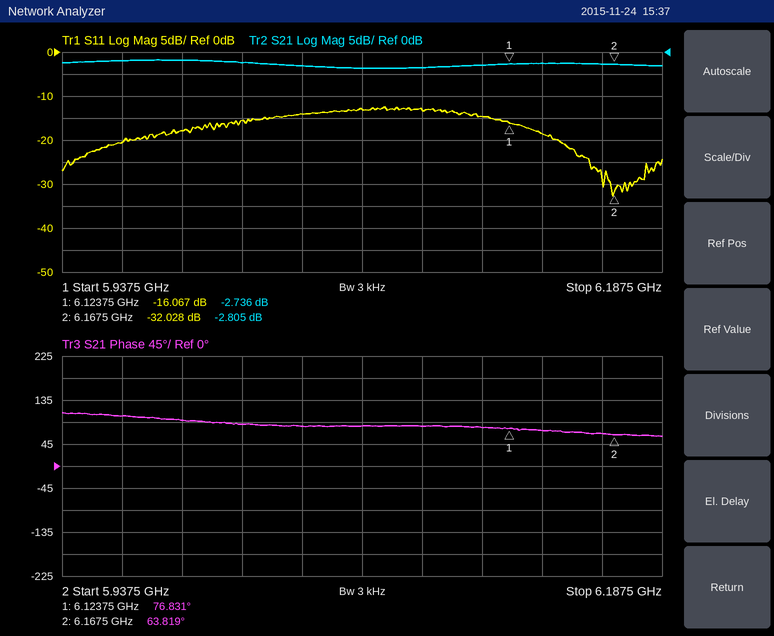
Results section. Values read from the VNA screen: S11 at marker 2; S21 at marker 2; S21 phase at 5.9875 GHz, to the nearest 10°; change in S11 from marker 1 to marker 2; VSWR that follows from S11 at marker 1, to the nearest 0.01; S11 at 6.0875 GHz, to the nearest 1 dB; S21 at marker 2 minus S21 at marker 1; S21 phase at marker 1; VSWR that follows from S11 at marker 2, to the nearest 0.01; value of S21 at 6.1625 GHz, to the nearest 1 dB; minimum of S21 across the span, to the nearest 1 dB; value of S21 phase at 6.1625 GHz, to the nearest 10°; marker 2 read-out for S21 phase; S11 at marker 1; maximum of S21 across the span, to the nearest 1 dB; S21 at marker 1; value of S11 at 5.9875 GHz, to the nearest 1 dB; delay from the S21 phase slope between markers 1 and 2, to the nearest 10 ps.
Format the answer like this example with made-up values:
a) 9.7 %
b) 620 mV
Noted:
a) -32.028 dB
b) -2.805 dB
c) 90°
d) -15.961 dB
e) 1.37
f) -13 dB
g) -0.069 dB
h) 76.831°
i) 1.05
j) -3 dB
k) -4 dB
l) 70°
m) 63.819°
n) -16.067 dB
o) -2 dB
p) -2.736 dB
q) -18 dB
r) 830 ps
